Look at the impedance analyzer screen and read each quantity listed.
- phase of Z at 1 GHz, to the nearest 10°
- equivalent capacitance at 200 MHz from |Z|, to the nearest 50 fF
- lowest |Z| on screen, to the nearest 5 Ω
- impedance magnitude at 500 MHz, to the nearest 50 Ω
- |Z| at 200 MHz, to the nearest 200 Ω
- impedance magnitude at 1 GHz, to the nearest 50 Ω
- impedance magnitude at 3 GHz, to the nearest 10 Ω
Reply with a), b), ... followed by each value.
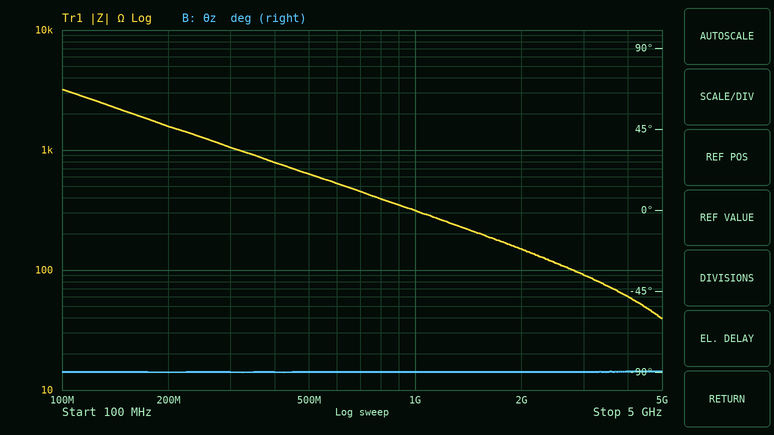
a) -90°
b) 500 fF
c) 40 Ω
d) 650 Ω
e) 1.6 kΩ
f) 300 Ω
g) 90 Ω
